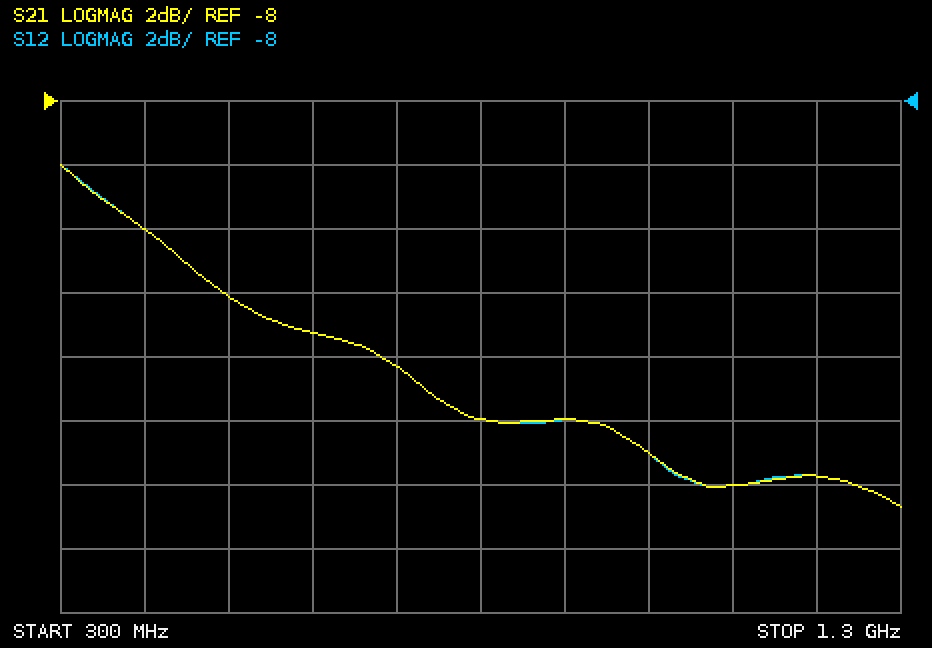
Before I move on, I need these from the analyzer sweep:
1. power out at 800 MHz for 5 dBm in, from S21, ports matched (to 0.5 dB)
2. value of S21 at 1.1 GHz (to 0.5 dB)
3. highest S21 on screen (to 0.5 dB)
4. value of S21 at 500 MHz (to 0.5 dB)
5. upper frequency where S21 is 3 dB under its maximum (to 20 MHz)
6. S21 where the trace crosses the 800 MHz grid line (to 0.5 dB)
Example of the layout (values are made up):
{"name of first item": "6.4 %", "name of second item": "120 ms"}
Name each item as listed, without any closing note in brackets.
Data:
{"power out at 800 MHz for 5 dBm in, from S21, ports matched": "-13.0 dBm", "value of S21 at 1.1 GHz": "-20.0 dB", "highest S21 on screen": "-10.0 dB", "value of S21 at 500 MHz": "-14.0 dB", "upper frequency where S21 is 3 dB under its maximum": "440 MHz", "S21 where the trace crosses the 800 MHz grid line": "-18.0 dB"}
